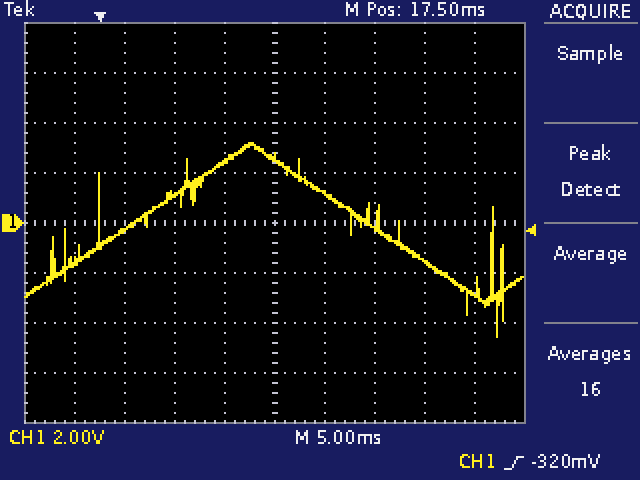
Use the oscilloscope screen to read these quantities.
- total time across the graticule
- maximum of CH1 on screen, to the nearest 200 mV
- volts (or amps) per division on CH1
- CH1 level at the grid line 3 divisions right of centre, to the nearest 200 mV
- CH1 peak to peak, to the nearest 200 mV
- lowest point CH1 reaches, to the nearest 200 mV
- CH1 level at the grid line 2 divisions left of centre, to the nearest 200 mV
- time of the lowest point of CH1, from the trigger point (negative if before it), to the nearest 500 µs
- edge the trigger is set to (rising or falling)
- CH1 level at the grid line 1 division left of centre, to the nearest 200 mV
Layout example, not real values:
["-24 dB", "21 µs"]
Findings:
["50 ms", "3.2 V", "2 V", "-1.6 V", "7.8 V", "-4.6 V", "1.2 V", "+40.0 ms", "rising", "2.4 V"]
